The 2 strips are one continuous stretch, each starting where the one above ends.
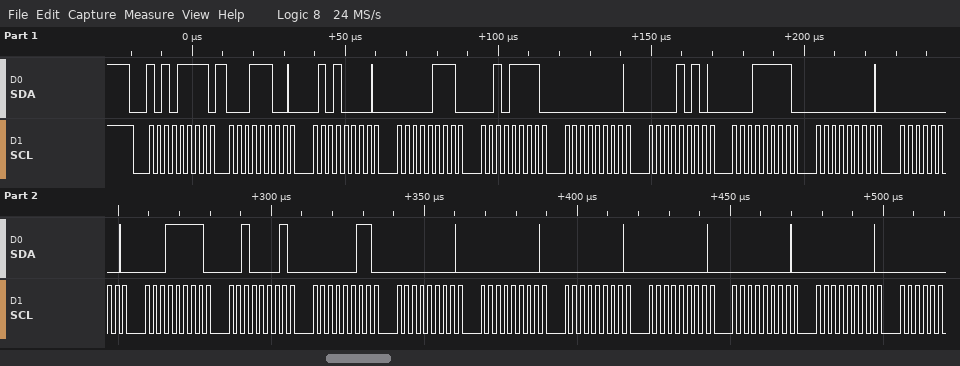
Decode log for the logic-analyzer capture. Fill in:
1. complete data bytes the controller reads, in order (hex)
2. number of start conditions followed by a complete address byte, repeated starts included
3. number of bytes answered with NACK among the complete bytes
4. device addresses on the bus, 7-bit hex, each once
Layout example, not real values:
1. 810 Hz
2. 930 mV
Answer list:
1. 1C 50 07 2F 00 0A 1F 00 00 1F 21 03 00 00 00 00 00 00
2. 1
3. 0
4. 0x57
